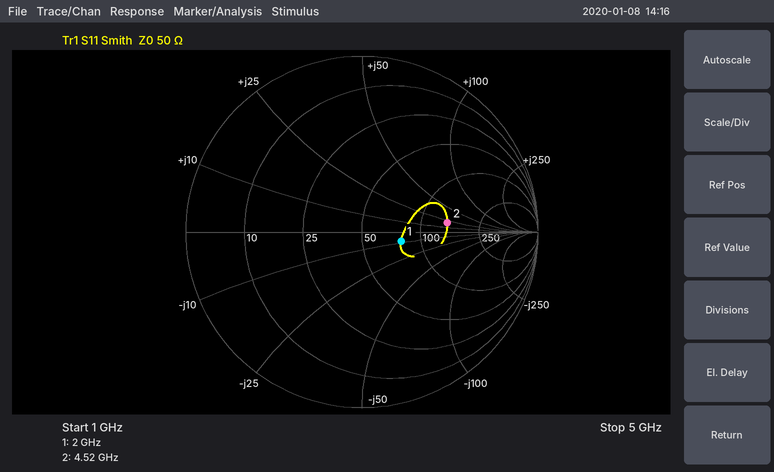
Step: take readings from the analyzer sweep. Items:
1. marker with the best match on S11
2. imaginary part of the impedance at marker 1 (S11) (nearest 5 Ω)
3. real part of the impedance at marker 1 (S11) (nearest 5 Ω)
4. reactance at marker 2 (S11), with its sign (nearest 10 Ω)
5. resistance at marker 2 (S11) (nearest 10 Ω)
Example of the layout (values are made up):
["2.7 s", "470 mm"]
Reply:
["marker 1", "-10 Ω", "80 Ω", "+20 Ω", "140 Ω"]
